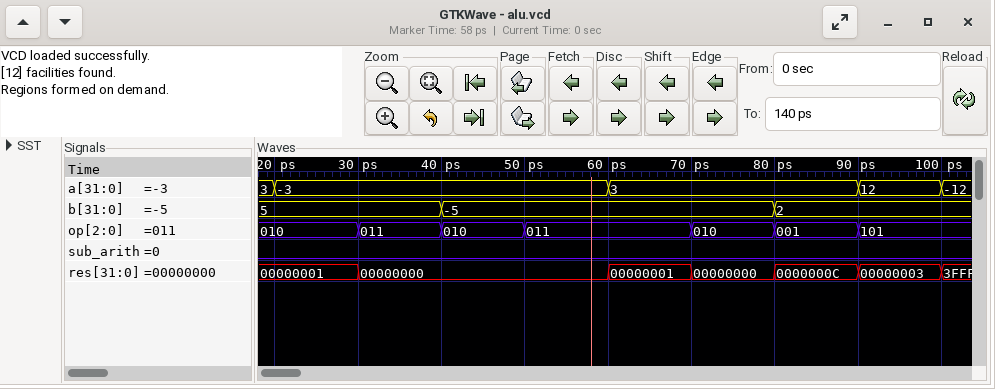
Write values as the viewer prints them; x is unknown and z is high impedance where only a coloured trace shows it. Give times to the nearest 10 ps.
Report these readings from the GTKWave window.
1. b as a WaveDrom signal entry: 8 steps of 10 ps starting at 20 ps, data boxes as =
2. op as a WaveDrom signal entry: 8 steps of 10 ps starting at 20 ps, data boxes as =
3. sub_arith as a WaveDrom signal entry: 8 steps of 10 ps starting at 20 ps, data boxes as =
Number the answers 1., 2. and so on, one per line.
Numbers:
1. {name: 'b', wave: '=.=...=.', data: '5 -5 2'}
2. {name: 'op', wave: '====.===', data: '010 011 010 011 010 001 101'}
3. {name: 'sub_arith', wave: '0.......'}
